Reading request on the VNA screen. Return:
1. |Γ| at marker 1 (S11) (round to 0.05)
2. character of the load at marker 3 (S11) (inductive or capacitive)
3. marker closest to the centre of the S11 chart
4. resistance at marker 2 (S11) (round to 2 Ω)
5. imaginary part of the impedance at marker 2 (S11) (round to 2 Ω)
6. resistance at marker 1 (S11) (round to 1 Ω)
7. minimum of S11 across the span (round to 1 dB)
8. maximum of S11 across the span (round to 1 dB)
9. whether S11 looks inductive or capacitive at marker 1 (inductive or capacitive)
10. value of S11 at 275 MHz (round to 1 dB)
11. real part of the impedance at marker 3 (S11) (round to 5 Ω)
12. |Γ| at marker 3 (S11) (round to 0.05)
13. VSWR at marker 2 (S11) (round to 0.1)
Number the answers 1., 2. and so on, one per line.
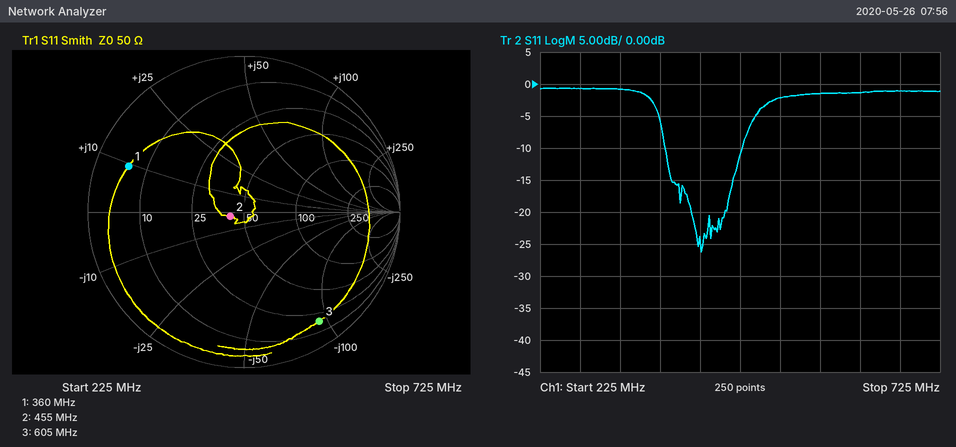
1. 0.80
2. capacitive
3. marker 2
4. 42 Ω
5. -2 Ω
6. 6 Ω
7. -26 dB
8. -1 dB
9. inductive
10. -1 dB
11. 20 Ω
12. 0.85
13. 1.2
